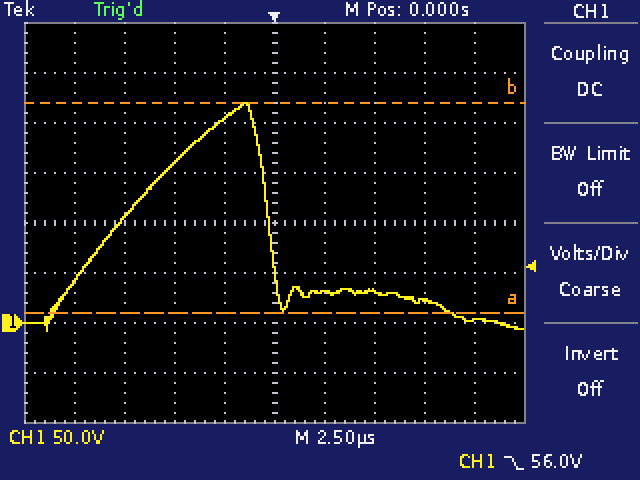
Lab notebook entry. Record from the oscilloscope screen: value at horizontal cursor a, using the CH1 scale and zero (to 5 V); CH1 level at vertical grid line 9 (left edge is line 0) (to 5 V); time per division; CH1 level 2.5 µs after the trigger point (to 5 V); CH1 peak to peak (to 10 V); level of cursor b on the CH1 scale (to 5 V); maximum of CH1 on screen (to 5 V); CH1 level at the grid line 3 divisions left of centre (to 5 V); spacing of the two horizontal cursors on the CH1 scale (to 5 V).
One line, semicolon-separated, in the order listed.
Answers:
10 V; 5 V; 2.5 µs; 30 V; 230 V; 220 V; 220 V; 105 V; 210 V
